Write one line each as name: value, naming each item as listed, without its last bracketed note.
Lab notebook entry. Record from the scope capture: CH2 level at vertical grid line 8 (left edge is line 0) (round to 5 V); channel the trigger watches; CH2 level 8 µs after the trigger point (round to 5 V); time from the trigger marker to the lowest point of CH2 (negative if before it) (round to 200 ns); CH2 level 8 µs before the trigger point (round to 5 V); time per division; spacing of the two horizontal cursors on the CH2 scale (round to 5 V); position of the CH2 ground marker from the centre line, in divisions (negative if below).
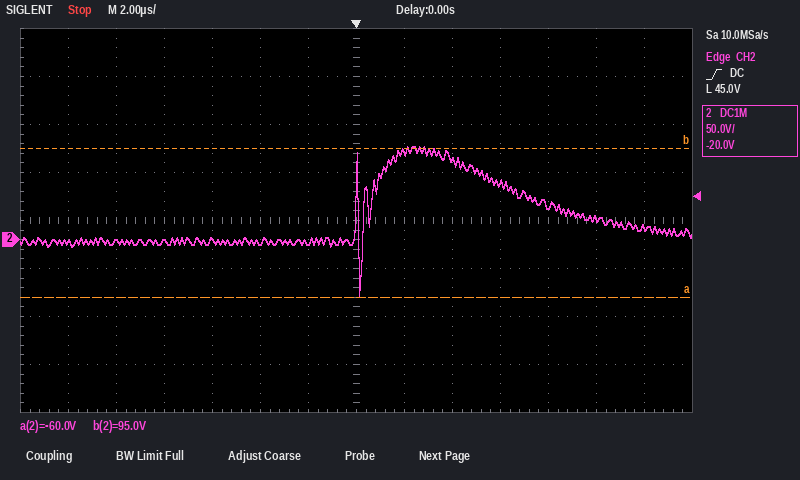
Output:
CH2 level at vertical grid line 8 (left edge is line 0): 90 V
channel the trigger watches: CH2
CH2 level 8 µs after the trigger point: 35 V
time from the trigger marker to the lowest point of CH2 (negative if before it): +200 ns
CH2 level 8 µs before the trigger point: 0 V
time per division: 2 µs
spacing of the two horizontal cursors on the CH2 scale: 155 V
position of the CH2 ground marker from the centre line, in divisions: -0.4 div
